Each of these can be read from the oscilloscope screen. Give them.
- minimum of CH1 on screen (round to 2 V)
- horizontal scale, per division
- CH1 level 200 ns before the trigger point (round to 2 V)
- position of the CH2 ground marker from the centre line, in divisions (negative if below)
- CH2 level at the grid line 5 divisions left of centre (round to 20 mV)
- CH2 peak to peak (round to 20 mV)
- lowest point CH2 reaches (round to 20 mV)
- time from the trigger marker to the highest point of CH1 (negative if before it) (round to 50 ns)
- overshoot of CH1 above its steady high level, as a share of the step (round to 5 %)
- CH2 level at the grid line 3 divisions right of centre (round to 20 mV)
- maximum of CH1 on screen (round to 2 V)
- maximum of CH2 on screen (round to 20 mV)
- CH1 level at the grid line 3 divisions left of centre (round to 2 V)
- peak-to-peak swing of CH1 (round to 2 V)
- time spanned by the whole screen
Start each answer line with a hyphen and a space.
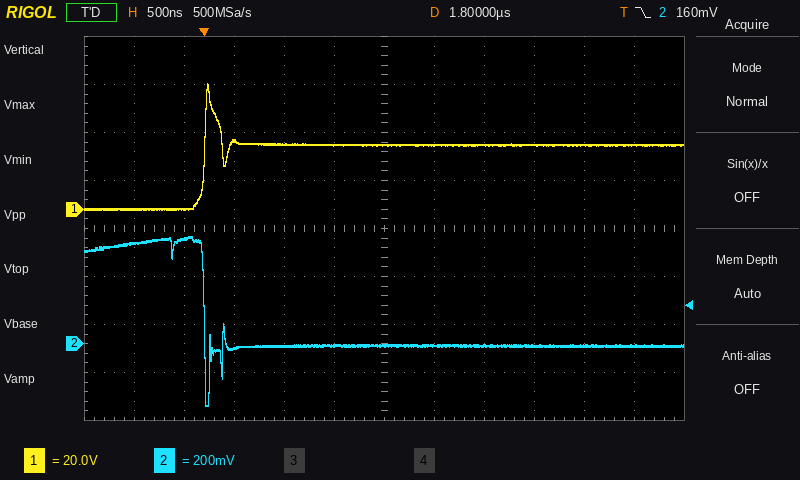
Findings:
- 0 V
- 500 ns
- 0 V
- -2.4 div
- 420 mV
- 700 mV
- -260 mV
- +50 ns
- 95 %
- 0 mV
- 52 V
- 440 mV
- 28 V
- 52 V
- 6 µs
